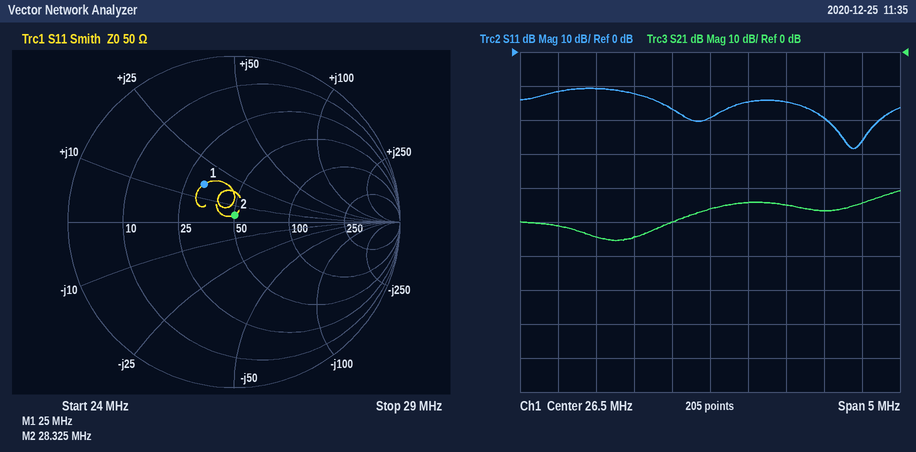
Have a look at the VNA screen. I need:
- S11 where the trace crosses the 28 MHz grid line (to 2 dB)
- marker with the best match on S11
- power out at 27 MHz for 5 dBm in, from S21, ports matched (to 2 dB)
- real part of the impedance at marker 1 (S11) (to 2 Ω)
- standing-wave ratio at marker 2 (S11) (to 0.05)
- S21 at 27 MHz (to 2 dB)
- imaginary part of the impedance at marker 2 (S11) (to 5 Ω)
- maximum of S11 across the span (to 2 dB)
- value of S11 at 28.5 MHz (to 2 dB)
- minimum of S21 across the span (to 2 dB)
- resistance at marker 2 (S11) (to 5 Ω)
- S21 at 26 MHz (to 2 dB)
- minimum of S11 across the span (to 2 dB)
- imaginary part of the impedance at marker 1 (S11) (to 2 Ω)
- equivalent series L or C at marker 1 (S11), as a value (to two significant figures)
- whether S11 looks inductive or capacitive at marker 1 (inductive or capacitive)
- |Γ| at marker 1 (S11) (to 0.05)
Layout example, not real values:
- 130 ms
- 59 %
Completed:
- -20 dB
- marker 2
- -40 dBm
- 32 Ω
- 1.10
- -44 dB
- +5 Ω
- -10 dB
- -26 dB
- -56 dB
- 50 Ω
- -50 dB
- -28 dB
- +16 Ω
- 100 nH
- inductive
- 0.30
